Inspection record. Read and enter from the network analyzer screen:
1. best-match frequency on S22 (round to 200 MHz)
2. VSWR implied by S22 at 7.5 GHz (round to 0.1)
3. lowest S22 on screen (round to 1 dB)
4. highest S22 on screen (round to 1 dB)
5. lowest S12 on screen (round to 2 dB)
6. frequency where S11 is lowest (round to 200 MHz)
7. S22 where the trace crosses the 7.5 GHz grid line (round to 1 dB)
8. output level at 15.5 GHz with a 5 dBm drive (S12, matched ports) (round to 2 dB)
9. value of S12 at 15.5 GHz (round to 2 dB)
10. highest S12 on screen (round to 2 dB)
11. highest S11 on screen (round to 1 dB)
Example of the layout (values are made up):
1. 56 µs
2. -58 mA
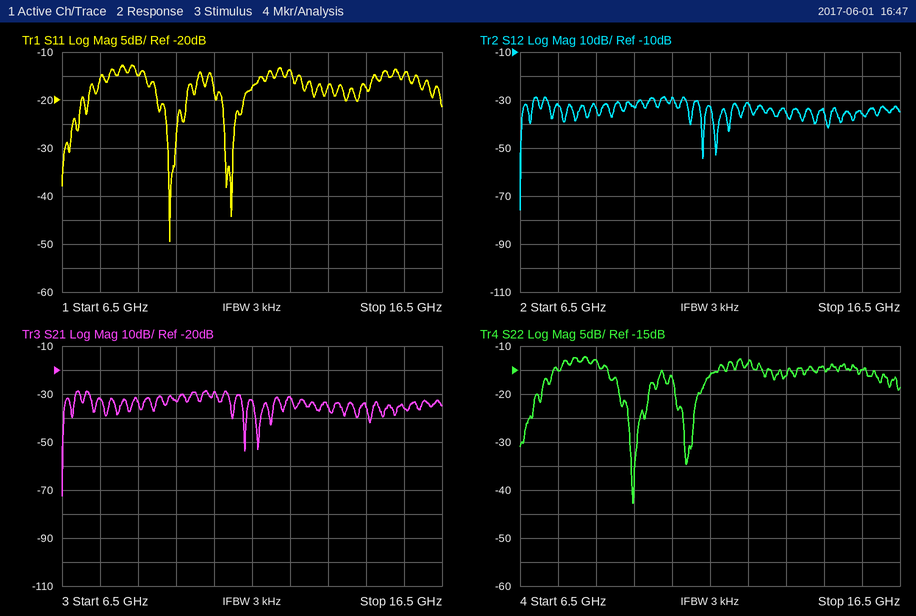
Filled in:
1. 9.4 GHz
2. 1.4
3. -43 dB
4. -12 dB
5. -76 dB
6. 9.4 GHz
7. -15 dB
8. -30 dBm
9. -36 dB
10. -28 dB
11. -13 dB
